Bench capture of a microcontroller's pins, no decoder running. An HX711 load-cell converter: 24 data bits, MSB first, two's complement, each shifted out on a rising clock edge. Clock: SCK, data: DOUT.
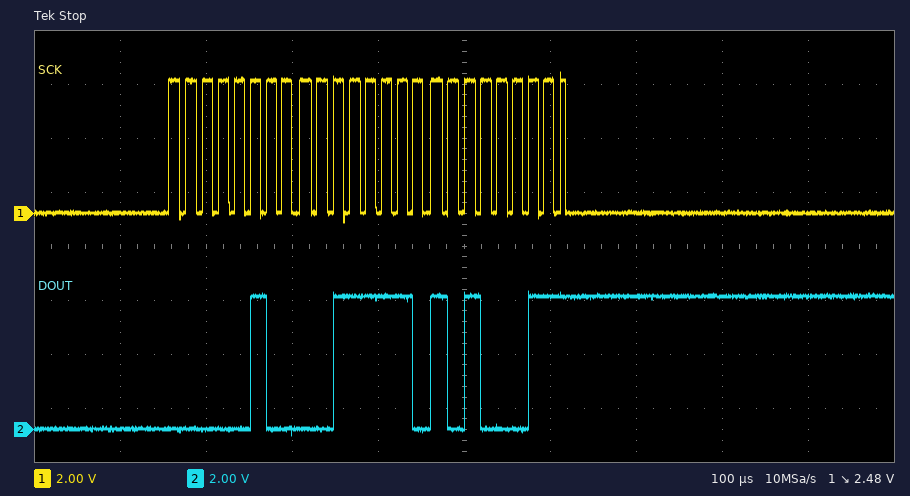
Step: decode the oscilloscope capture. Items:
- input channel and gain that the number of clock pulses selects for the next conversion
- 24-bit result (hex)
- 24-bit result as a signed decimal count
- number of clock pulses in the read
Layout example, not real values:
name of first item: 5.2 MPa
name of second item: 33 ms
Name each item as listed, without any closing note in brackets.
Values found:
input channel and gain that the number of clock pulses selects for the next conversion: channel A, gain 128
24-bit result: 0x043EA3
24-bit result as a signed decimal count: 278179
number of clock pulses in the read: 25
